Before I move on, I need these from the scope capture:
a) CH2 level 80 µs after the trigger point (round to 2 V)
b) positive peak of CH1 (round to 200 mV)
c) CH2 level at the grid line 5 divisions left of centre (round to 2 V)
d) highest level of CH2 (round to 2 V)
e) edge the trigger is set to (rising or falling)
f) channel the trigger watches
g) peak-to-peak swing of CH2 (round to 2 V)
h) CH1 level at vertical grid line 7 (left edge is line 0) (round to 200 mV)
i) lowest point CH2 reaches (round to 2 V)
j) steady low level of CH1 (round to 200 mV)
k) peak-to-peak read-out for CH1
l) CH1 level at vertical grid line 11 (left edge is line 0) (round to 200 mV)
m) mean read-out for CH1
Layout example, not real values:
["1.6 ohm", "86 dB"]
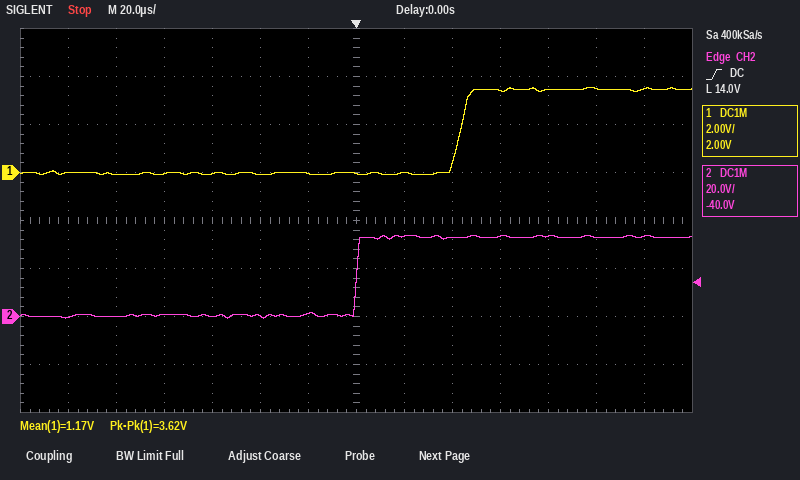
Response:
["34 V", "3.6 V", "0 V", "34 V", "rising", "CH2", "34 V", "0.0 V", "0 V", "0.0 V", "3.62 V", "3.4 V", "1.17 V"]
